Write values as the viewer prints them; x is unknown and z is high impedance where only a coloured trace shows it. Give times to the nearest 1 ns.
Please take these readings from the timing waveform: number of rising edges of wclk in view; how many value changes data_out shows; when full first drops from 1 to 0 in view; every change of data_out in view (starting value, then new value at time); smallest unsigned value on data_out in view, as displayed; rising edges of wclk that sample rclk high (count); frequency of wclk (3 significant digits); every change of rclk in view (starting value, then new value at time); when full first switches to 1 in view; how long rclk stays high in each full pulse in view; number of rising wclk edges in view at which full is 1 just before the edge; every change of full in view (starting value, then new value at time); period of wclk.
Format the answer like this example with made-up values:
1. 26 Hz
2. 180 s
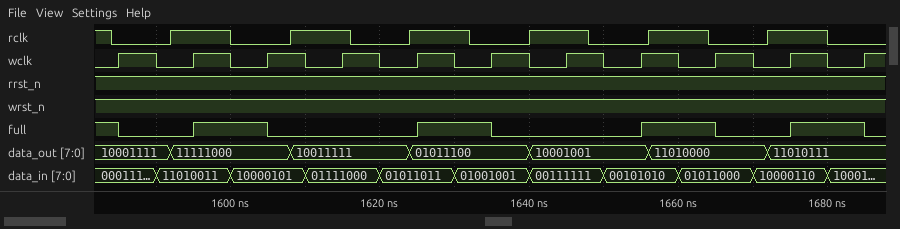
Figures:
1. 11
2. 6
3. 1585 ns
4. 10001111, 11111000 at 1592 ns, 10011111 at 1608 ns, 01011100 at 1624 ns, 10001001 at 1640 ns, 11010000 at 1656 ns, 11010111 at 1672 ns
5. 01011100
6. 5
7. 100 MHz
8. 1, 0 at 1584 ns, 1 at 1592 ns, 0 at 1600 ns, 1 at 1608 ns, 0 at 1616 ns, 1 at 1624 ns, 0 at 1632 ns, 1 at 1640 ns, 0 at 1648 ns, 1 at 1656 ns, 0 at 1664 ns, 1 at 1672 ns, 0 at 1680 ns
9. 1595 ns
10. 8 ns, 8 ns, 8 ns, 8 ns, 8 ns, 8 ns
11. 5
12. 1, 0 at 1585 ns, 1 at 1595 ns, 0 at 1605 ns, 1 at 1625 ns, 0 at 1635 ns, 1 at 1655 ns, 0 at 1665 ns, 1 at 1675 ns, 0 at 1685 ns
13. 10 ns
